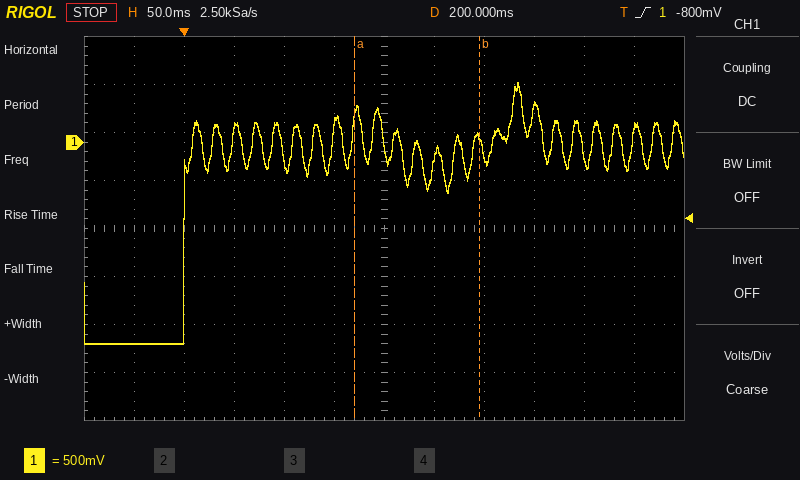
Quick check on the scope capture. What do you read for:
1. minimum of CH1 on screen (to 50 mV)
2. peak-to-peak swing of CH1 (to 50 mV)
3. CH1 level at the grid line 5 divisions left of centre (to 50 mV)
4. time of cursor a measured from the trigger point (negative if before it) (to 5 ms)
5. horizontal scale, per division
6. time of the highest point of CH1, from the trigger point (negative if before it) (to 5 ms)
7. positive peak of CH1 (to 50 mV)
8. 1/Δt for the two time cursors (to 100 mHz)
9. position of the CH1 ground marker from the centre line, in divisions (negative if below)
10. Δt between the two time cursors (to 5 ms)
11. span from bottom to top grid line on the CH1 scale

-2.10 V
2.70 V
-2.10 V
+170 ms
50 ms
+335 ms
600 mV
8.0 Hz
+1.8 div
125 ms
4 V
